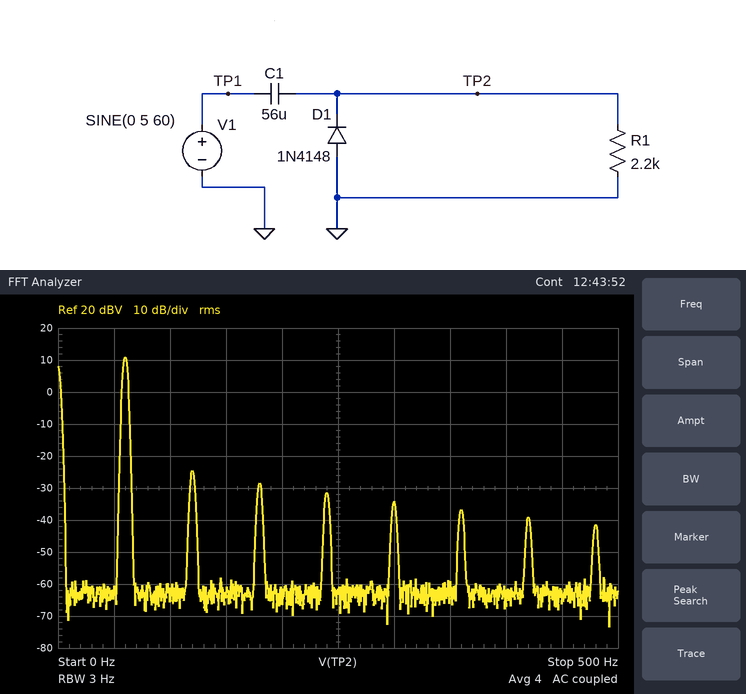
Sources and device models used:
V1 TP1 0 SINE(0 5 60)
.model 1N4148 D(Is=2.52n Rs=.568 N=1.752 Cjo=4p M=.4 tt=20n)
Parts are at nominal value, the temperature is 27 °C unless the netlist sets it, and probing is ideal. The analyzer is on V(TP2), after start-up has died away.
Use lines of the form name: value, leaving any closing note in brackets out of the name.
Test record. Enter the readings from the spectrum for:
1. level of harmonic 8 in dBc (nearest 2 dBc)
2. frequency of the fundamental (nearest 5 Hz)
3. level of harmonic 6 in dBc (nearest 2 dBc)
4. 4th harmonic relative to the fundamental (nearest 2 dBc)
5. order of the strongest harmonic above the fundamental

level of harmonic 8 in dBc: -52 dBc
frequency of the fundamental: 60 Hz
level of harmonic 6 in dBc: -48 dBc
4th harmonic relative to the fundamental: -42 dBc
order of the strongest harmonic above the fundamental: 2
